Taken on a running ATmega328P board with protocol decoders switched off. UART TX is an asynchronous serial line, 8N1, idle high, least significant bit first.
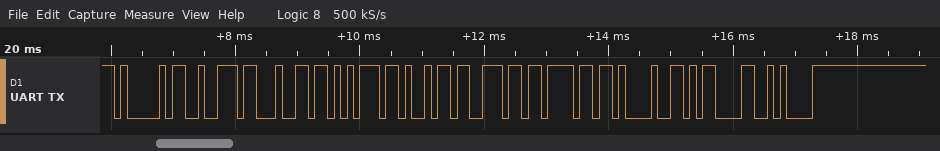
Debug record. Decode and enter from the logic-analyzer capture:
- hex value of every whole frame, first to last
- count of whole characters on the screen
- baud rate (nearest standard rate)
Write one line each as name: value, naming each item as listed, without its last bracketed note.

hex value of every whole frame, first to last: 0x41 0x72 0x64 0x75 0x69 0x6E 0x6F 0x21 0x0D 0x0A
count of whole characters on the screen: 10
baud rate: 9600 baud
